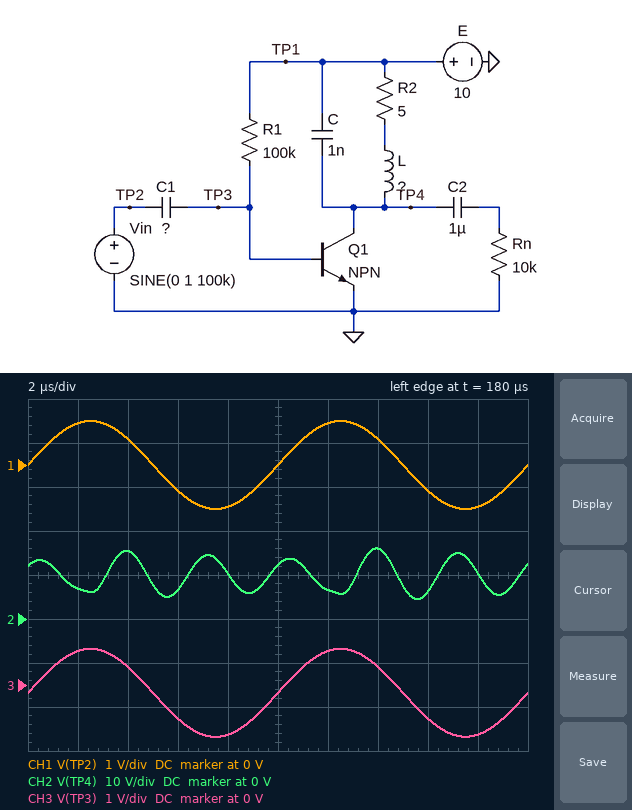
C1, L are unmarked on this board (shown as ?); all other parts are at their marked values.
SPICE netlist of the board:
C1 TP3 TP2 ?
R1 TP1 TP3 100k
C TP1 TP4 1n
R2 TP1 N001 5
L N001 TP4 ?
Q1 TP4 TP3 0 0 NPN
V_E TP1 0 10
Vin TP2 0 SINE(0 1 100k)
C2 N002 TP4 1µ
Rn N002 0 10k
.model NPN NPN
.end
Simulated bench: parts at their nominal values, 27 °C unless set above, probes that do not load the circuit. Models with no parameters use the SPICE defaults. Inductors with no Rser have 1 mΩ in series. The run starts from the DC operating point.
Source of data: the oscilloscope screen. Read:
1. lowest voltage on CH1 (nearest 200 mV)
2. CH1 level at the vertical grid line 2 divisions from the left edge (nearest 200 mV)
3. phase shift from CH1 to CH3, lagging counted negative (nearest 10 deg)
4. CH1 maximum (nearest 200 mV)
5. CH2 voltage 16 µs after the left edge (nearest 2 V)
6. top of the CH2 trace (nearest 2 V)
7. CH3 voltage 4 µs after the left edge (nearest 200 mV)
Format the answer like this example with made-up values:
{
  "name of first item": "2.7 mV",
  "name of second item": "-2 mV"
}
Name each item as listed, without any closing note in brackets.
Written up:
{
  "lowest voltage on CH1": "-1.0 V",
  "CH1 level at the vertical grid line 2 divisions from the left edge": "600 mV",
  "phase shift from CH1 to CH3, lagging counted negative": "0 deg",
  "CH1 maximum": "1.0 V",
  "CH2 voltage 16 µs after the left edge": "6 V",
  "top of the CH2 trace": "16 V",
  "CH3 voltage 4 µs after the left edge": "400 mV"
}
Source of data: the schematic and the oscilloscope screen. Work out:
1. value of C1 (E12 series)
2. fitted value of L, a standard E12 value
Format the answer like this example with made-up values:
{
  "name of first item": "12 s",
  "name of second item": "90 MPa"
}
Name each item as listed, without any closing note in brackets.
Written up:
{
  "value of C1": "390 nF",
  "fitted value of L, a standard E12 value": "270 µH"
}
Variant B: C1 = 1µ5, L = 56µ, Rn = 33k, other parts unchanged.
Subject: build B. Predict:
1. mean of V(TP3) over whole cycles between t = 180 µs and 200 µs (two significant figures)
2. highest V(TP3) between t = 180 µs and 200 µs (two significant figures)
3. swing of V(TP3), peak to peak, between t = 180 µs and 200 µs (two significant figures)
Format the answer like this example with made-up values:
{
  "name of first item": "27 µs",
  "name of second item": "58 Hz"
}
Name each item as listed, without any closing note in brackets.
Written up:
{
  "mean of V(TP3) over whole cycles between t = 180 µs and 200 µs": "-150 mV",
  "highest V(TP3) between t = 180 µs and 200 µs": "850 mV",
  "swing of V(TP3), peak to peak, between t = 180 µs and 200 µs": "2.0 V"
}
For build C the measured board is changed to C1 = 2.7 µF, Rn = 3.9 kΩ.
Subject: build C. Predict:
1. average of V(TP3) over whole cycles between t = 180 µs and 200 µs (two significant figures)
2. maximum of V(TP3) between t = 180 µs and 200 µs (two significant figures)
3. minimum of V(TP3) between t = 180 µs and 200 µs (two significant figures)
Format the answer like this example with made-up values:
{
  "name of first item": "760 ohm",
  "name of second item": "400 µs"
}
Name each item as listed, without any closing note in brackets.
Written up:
{
  "average of V(TP3) over whole cycles between t = 180 µs and 200 µs": "-140 mV",
  "maximum of V(TP3) between t = 180 µs and 200 µs": "860 mV",
  "minimum of V(TP3) between t = 180 µs and 200 µs": "-1.1 V"
}
